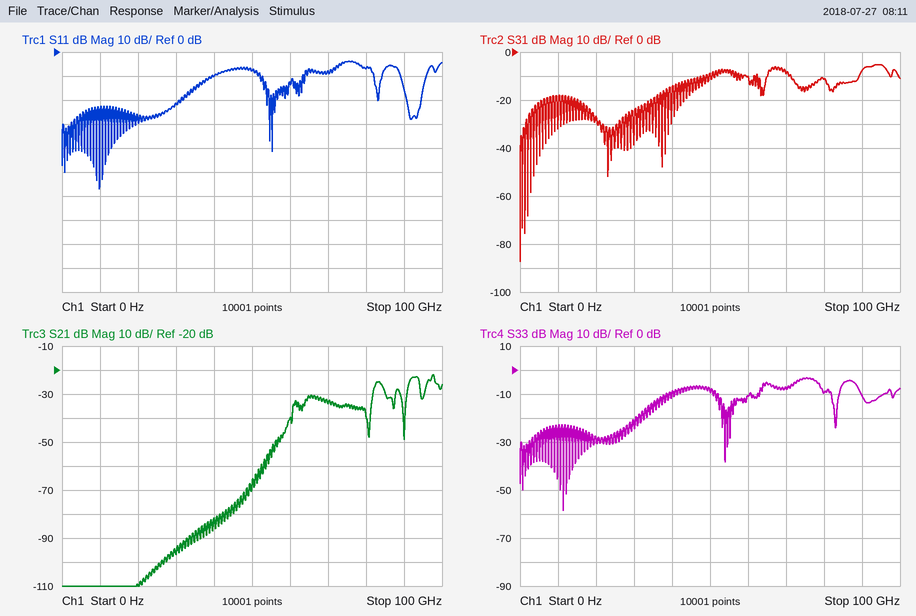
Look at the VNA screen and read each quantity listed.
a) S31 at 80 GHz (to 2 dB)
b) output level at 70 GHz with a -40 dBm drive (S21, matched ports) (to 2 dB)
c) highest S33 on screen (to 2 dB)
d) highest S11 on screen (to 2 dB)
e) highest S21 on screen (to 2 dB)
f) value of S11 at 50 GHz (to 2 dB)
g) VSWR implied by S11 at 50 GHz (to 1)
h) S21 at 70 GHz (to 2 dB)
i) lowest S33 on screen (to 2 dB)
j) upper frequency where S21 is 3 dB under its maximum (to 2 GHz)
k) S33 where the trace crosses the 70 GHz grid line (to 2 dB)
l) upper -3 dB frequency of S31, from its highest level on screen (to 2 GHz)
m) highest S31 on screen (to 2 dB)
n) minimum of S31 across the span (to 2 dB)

-12 dB
-74 dBm
-4 dB
-4 dB
-22 dB
-8 dB
2
-34 dB
-58 dB
98 GHz
-8 dB
96 GHz
-6 dB
-88 dB
